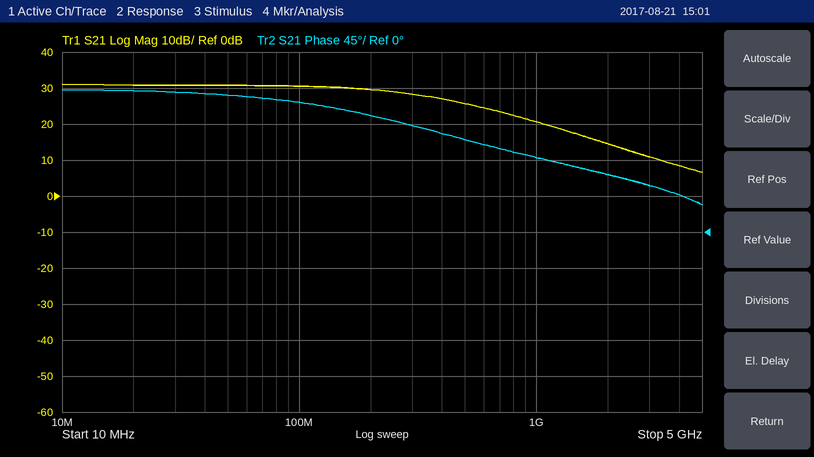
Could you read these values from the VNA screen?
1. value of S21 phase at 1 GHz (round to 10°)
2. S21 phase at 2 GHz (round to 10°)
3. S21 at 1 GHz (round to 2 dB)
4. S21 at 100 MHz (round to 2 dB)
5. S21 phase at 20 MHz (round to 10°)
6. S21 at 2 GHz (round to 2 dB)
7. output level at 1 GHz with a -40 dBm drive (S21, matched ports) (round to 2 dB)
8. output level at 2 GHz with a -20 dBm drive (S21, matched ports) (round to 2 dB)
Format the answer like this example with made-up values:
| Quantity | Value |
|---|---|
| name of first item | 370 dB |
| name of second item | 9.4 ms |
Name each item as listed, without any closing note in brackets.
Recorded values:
| Quantity | Value |
|---|---|
| value of S21 phase at 1 GHz | 90° |
| S21 phase at 2 GHz | 70° |
| S21 at 1 GHz | 20 dB |
| S21 at 100 MHz | 30 dB |
| S21 phase at 20 MHz | 180° |
| S21 at 2 GHz | 14 dB |
| output level at 1 GHz with a -40 dBm drive (S21, matched ports) | -20 dBm |
| output level at 2 GHz with a -20 dBm drive (S21, matched ports) | -6 dBm |
